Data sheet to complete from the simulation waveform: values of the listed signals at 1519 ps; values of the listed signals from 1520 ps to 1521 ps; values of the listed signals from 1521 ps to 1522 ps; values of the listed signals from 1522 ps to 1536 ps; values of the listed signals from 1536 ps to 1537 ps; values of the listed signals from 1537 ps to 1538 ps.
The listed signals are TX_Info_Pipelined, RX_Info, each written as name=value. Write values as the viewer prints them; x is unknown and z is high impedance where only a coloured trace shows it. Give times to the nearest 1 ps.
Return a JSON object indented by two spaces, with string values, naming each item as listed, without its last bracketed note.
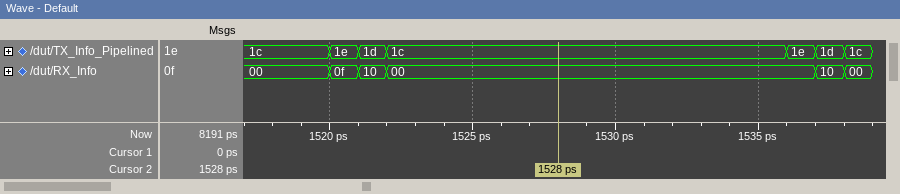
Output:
{
  "values of the listed signals at 1519 ps": "TX_Info_Pipelined=1c, RX_Info=00",
  "values of the listed signals from 1520 ps to 1521 ps": "TX_Info_Pipelined=1e, RX_Info=0f",
  "values of the listed signals from 1521 ps to 1522 ps": "TX_Info_Pipelined=1d, RX_Info=10",
  "values of the listed signals from 1522 ps to 1536 ps": "TX_Info_Pipelined=1c, RX_Info=00",
  "values of the listed signals from 1536 ps to 1537 ps": "TX_Info_Pipelined=1e, RX_Info=00",
  "values of the listed signals from 1537 ps to 1538 ps": "TX_Info_Pipelined=1d, RX_Info=10"
}
